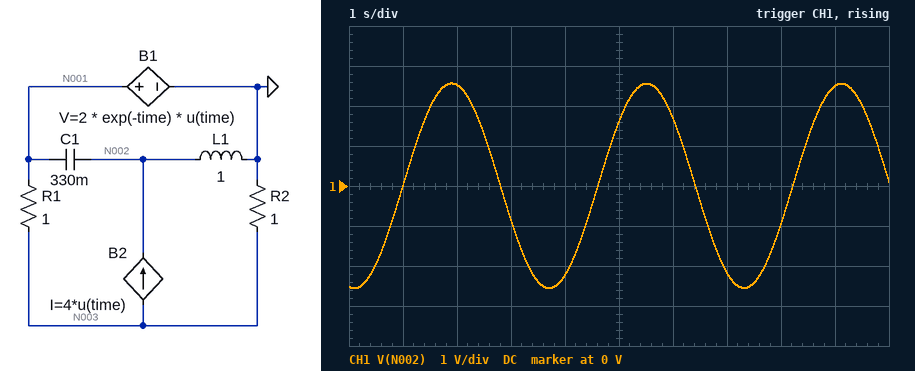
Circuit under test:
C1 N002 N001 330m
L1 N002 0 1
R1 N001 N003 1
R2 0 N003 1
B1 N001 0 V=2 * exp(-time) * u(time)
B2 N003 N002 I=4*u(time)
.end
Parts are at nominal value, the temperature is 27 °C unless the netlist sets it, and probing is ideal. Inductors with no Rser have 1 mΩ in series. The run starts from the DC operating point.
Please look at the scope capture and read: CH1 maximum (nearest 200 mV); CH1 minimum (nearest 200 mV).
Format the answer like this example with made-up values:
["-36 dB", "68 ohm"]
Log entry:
["2.6 V", "-2.6 V"]
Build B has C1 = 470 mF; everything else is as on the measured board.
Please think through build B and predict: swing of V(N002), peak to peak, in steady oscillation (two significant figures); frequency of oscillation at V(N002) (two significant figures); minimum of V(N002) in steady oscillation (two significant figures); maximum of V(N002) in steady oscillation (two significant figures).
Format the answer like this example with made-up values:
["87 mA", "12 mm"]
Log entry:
["3.9 V", "230 mHz", "-1.9 V", "1.9 V"]
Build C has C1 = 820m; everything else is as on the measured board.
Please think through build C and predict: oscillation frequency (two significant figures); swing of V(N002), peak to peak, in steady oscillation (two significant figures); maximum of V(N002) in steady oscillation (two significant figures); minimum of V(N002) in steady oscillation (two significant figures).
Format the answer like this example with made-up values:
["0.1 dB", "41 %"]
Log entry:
["180 mHz", "2.3 V", "1.2 V", "-1.2 V"]
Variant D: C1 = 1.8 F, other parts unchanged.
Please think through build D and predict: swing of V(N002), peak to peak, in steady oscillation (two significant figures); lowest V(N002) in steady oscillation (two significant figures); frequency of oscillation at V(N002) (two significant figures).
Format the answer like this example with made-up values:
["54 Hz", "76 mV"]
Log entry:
["1.2 V", "-580 mV", "120 mHz"]
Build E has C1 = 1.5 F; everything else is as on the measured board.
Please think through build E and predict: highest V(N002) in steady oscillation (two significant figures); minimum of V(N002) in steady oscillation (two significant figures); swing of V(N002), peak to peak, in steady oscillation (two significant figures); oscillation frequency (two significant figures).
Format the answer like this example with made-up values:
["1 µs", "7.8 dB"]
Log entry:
["660 mV", "-650 mV", "1.3 V", "130 mHz"]
